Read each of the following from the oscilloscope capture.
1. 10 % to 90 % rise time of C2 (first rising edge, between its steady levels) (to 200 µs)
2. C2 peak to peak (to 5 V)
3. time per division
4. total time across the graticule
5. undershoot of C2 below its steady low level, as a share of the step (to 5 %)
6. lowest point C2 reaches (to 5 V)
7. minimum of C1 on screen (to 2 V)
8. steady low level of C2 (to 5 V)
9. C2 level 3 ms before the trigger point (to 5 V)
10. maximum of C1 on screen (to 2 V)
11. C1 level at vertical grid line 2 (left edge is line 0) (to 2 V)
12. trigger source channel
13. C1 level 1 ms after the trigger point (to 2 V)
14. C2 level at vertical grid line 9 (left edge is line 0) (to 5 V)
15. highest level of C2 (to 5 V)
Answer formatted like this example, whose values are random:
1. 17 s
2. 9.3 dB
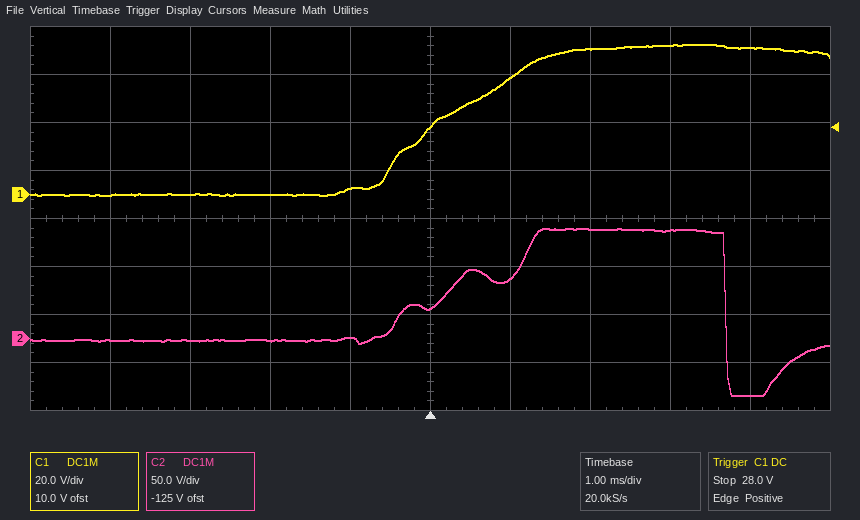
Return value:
1. 1.8 ms
2. 175 V
3. 1 ms
4. 10 ms
5. 50 %
6. -60 V
7. 0 V
8. 0 V
9. 0 V
10. 62 V
11. 0 V
12. C1
13. 48 V
14. -60 V
15. 115 V
